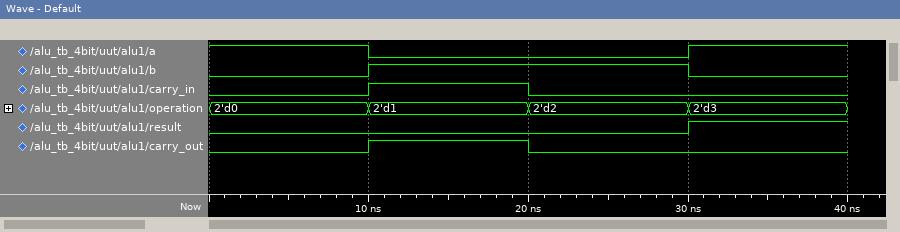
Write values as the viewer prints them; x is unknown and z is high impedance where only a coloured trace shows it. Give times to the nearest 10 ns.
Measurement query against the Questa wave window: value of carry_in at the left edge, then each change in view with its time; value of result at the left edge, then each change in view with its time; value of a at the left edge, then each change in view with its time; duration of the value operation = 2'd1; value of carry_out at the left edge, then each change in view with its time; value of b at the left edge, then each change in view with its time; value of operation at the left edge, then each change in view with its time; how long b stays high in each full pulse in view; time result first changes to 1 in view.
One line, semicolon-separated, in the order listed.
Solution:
0, 1 at 10 ns, 0 at 20 ns; 0, 1 at 30 ns; 1, 0 at 10 ns, 1 at 30 ns; 10 ns; 0, 1 at 10 ns, 0 at 20 ns; 0, 1 at 10 ns, 0 at 30 ns; 2'd0, 2'd1 at 10 ns, 2'd2 at 20 ns, 2'd3 at 30 ns; 20 ns; 30 ns
